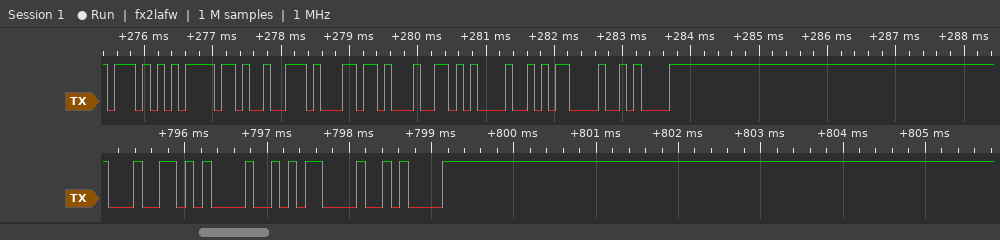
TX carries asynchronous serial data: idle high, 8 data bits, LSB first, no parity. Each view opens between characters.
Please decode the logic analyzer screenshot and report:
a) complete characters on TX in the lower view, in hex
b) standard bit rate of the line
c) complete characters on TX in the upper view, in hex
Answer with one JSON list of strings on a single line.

["64, 21, 0D, 0A", "9600 baud", "57, 6F, 72, 6C, 64, 21, 0D, 0A"]
